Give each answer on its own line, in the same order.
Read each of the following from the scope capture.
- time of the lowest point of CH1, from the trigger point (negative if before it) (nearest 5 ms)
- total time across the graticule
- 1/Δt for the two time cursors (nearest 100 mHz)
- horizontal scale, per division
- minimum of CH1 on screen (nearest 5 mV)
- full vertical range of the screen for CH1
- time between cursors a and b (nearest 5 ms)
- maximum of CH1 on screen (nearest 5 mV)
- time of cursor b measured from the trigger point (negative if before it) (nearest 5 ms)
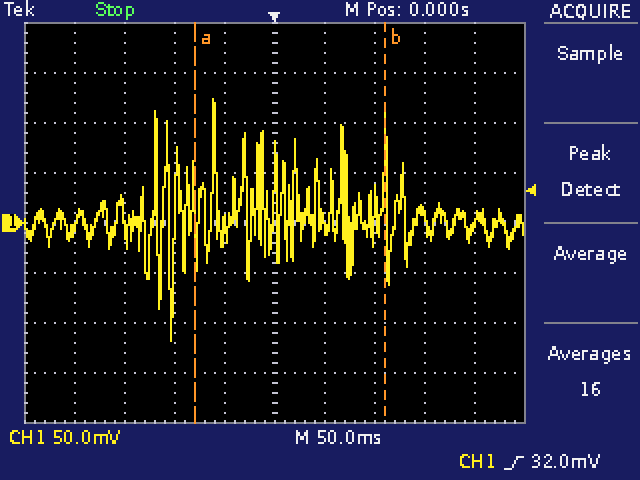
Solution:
-105 ms
500 ms
5.3 Hz
50 ms
-120 mV
400 mV
190 ms
125 mV
+110 ms
